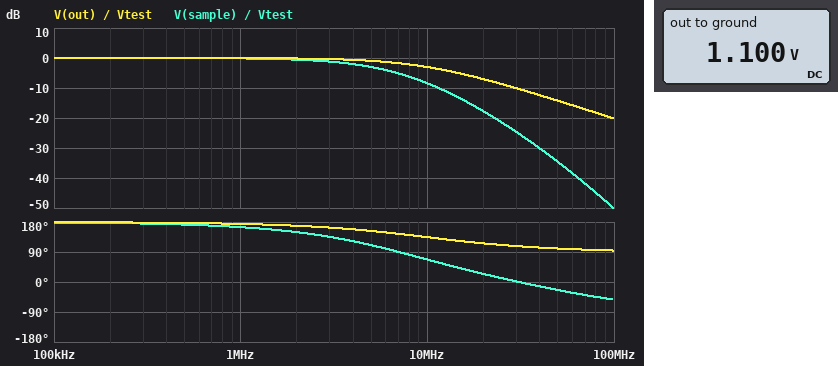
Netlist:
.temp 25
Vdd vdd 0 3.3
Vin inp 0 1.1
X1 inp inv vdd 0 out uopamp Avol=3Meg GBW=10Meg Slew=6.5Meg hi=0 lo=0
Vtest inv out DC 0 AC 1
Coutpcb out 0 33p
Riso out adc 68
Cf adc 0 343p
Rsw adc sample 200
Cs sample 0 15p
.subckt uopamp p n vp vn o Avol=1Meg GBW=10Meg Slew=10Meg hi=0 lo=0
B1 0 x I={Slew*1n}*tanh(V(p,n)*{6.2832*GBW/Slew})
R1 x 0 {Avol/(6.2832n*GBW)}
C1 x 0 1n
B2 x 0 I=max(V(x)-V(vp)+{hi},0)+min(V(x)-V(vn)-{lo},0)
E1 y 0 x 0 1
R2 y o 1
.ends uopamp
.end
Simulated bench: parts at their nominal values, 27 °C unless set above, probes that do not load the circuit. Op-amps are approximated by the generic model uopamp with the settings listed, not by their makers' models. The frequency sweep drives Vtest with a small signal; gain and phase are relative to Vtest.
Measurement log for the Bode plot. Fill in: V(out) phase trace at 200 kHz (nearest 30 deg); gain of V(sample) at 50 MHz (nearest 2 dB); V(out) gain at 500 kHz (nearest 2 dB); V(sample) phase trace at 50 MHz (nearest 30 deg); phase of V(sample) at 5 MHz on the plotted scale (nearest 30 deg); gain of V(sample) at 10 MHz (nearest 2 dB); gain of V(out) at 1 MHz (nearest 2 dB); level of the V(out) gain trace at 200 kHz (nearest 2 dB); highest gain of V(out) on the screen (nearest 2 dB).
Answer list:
180 deg
-34 dB
0 dB
-30 deg
120 deg
-8 dB
0 dB
0 dB
0 dB
